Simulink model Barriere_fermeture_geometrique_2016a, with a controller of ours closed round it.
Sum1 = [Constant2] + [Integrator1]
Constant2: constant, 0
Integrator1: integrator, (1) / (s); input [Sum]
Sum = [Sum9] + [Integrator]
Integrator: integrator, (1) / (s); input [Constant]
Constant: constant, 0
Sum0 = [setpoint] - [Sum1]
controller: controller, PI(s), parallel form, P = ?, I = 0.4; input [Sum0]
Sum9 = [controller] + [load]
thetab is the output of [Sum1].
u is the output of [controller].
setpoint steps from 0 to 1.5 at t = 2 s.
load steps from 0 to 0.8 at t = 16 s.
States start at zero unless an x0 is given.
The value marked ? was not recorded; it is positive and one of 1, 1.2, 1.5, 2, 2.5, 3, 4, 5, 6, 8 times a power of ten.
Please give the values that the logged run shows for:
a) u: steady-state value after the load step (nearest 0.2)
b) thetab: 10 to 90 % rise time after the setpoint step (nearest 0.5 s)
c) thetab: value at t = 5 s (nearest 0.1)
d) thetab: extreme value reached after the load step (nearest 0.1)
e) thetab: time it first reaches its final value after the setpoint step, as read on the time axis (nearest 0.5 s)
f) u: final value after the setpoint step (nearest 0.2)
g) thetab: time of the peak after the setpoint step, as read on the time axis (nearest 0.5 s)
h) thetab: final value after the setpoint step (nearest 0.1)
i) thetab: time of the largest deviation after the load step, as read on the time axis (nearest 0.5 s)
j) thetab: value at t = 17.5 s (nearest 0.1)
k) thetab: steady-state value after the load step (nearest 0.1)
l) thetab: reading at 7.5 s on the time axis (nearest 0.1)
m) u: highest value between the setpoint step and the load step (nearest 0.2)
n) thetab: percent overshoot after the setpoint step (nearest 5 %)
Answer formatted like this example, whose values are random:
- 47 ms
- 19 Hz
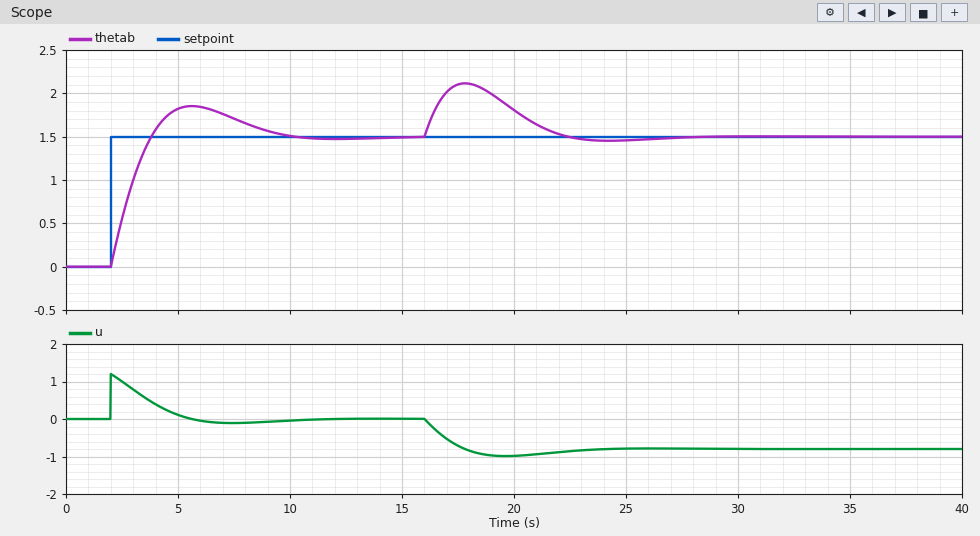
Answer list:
- -0.8
- 1.5 s
- 1.8
- 2.1
- 4.0 s
- 0.0
- 5.5 s
- 1.5
- 18.0 s
- 2.1
- 1.5
- 1.7
- 1.2
- 25 %
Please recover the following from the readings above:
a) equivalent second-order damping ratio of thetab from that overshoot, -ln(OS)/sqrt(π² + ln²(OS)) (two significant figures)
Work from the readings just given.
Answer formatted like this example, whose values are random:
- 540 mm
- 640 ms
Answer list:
- 0.40
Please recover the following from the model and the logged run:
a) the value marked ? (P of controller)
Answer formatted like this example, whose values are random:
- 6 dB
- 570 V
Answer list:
- 0.8
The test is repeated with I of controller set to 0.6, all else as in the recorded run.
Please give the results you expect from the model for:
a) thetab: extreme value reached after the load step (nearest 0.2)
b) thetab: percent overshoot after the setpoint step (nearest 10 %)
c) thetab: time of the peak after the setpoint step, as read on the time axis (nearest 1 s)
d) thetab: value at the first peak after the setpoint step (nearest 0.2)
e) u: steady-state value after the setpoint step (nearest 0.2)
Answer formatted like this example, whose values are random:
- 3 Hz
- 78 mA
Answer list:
- 2.0
- 30 %
- 5 s
- 2.0
- 0.0
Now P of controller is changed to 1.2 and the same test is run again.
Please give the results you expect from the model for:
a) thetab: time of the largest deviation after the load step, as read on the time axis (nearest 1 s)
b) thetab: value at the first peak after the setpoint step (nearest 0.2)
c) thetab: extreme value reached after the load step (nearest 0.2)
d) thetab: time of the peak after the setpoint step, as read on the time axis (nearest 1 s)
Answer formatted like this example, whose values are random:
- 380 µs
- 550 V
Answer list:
- 18 s
- 1.8
- 2.0
- 5 s
